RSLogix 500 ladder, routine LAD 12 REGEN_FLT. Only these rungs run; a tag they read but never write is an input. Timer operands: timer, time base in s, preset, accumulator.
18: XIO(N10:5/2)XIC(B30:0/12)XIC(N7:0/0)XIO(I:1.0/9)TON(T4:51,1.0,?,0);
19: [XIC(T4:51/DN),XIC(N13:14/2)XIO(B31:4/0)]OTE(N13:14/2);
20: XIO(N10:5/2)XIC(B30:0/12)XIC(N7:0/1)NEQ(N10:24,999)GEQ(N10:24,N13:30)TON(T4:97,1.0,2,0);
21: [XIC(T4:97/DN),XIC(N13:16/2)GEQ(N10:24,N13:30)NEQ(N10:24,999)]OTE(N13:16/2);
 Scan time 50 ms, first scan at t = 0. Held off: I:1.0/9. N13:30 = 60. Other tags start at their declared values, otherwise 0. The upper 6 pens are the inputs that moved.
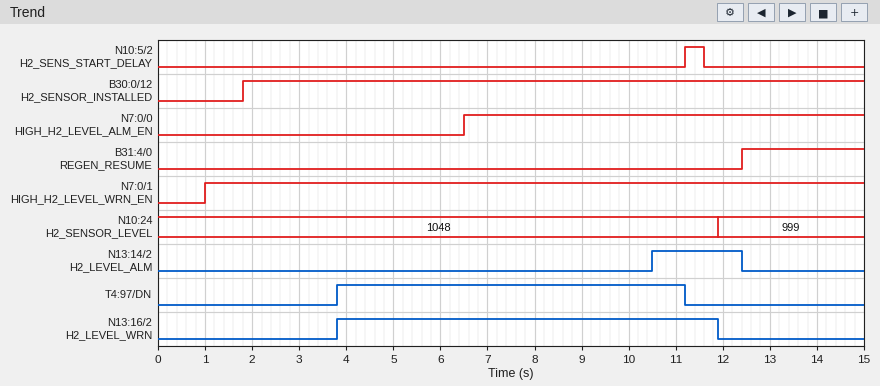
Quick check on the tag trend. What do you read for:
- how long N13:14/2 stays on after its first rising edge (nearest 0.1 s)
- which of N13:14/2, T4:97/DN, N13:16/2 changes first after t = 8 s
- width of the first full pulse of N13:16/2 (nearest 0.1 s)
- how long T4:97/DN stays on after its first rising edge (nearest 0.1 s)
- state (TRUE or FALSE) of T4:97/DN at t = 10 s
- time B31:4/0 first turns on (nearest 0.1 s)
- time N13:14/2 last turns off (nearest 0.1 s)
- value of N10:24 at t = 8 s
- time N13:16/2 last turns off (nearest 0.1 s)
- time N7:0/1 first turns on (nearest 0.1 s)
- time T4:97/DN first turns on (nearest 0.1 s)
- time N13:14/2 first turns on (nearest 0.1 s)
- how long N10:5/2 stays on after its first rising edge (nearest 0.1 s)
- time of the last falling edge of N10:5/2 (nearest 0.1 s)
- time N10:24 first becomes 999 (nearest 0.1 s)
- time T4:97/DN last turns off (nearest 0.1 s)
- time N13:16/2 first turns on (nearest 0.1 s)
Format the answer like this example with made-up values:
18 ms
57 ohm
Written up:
1.9 s
N13:14/2
8.1 s
7.4 s
TRUE
12.4 s
12.4 s
1048
11.9 s
1.0 s
3.8 s
10.5 s
0.4 s
11.6 s
11.9 s
11.2 s
3.8 s
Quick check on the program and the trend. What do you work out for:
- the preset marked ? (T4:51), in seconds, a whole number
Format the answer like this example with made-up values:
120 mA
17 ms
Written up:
4 s
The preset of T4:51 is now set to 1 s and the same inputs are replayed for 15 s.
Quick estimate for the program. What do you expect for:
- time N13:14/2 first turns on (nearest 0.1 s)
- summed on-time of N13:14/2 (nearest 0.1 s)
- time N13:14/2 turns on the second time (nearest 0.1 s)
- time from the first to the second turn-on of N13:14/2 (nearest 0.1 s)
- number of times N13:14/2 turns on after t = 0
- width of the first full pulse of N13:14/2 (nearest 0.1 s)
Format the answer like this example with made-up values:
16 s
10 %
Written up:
7.5 s
7.3 s
12.6 s
5.1 s
2
4.9 s
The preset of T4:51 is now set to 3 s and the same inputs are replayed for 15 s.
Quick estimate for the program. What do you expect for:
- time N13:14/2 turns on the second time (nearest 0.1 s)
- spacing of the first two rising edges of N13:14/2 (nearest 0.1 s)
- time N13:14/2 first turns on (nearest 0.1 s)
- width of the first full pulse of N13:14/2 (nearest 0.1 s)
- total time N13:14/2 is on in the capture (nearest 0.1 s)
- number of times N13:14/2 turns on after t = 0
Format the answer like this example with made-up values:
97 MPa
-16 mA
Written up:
14.6 s
5.1 s
9.5 s
2.9 s
3.3 s
2
